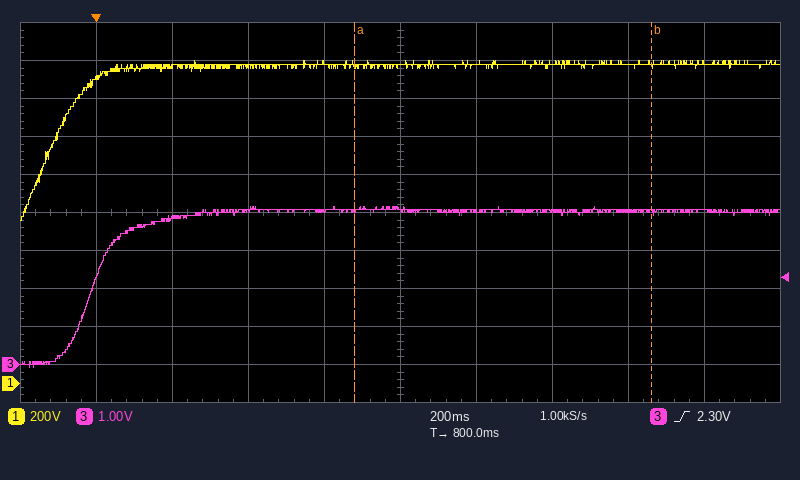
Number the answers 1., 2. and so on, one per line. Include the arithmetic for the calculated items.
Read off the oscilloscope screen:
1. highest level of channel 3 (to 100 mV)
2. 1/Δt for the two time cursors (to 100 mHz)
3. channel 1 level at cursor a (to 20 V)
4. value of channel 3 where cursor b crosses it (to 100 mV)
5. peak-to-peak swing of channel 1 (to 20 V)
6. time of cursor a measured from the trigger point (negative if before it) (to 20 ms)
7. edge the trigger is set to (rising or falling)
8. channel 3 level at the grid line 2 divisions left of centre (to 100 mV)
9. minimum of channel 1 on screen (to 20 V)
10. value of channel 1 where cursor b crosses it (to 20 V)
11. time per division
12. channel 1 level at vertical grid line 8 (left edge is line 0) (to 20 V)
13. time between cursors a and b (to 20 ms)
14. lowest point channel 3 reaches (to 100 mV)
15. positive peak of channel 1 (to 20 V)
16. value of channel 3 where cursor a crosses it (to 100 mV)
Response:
1. 4.2 V
2. 1 / 780 ms ≈ 1.3 Hz
3. 1.68 kV
4. 4.0 V
5. 1.70 kV − (860 V) = 840 V
6. +680 ms
7. rising
8. 4.1 V
9. 860 V
10. 1.68 kV
11. 200 ms
12. 1.68 kV
13. 780 ms
14. -100 mV
15. 1.70 kV
16. 4.0 V
